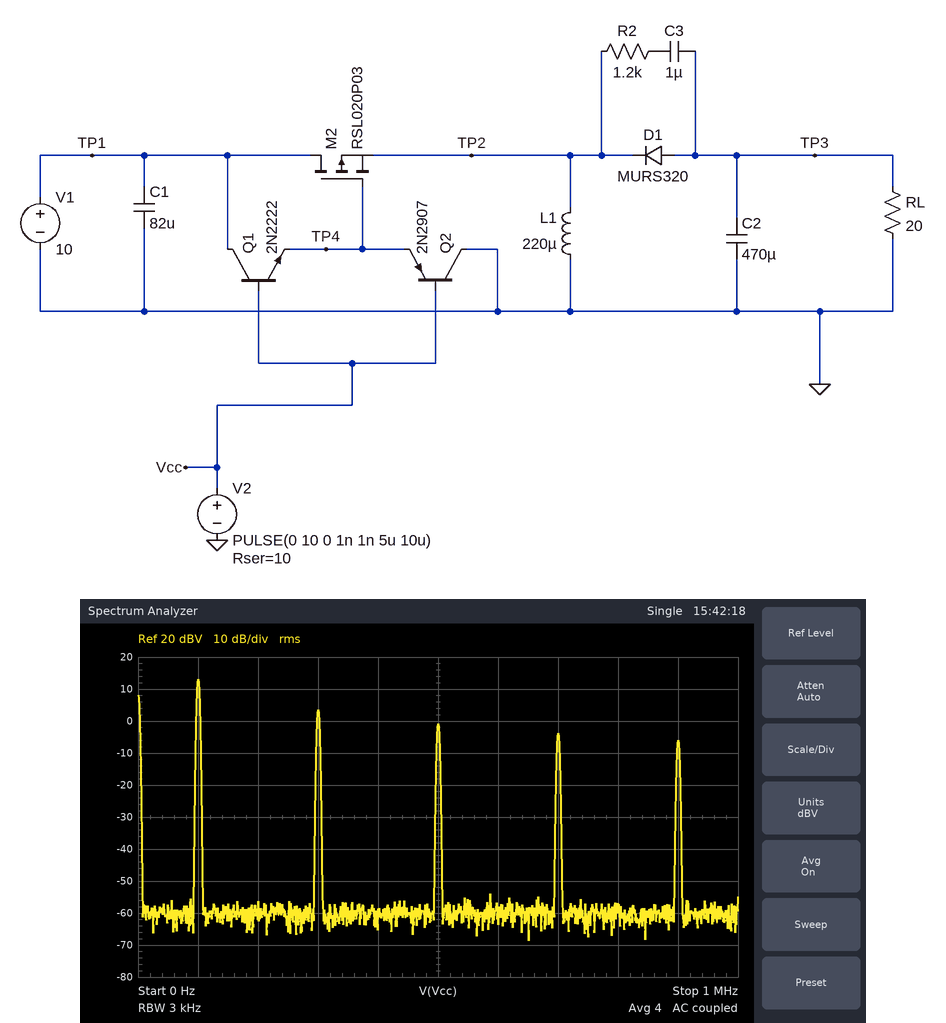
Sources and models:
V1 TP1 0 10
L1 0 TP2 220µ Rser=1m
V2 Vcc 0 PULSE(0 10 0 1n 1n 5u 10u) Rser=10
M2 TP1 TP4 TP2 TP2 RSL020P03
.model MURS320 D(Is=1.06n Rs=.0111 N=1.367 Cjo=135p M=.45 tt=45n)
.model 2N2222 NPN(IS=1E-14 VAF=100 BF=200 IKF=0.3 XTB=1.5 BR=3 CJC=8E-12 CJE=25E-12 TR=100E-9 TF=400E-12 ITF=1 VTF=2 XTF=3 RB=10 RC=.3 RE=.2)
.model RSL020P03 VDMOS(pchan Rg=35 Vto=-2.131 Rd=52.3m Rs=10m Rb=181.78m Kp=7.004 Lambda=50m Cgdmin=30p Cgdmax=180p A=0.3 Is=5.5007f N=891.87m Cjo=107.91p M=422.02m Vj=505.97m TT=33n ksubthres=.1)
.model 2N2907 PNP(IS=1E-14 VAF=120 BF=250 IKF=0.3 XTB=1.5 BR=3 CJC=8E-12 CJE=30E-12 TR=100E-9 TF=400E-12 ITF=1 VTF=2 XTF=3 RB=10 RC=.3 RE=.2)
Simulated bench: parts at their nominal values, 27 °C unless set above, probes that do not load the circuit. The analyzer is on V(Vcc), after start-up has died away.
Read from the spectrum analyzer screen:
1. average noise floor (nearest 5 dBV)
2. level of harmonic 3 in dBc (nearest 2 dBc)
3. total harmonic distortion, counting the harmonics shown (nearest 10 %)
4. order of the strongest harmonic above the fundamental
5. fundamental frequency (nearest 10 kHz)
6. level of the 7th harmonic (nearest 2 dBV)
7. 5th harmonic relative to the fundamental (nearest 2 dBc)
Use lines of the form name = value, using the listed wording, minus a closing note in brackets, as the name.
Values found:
average noise floor = -60 dBV
level of harmonic 3 in dBc = -10 dBc
total harmonic distortion, counting the harmonics shown = 40 %
order of the strongest harmonic above the fundamental = 3
fundamental frequency = 100 kHz
level of the 7th harmonic = -4 dBV
5th harmonic relative to the fundamental = -14 dBc
